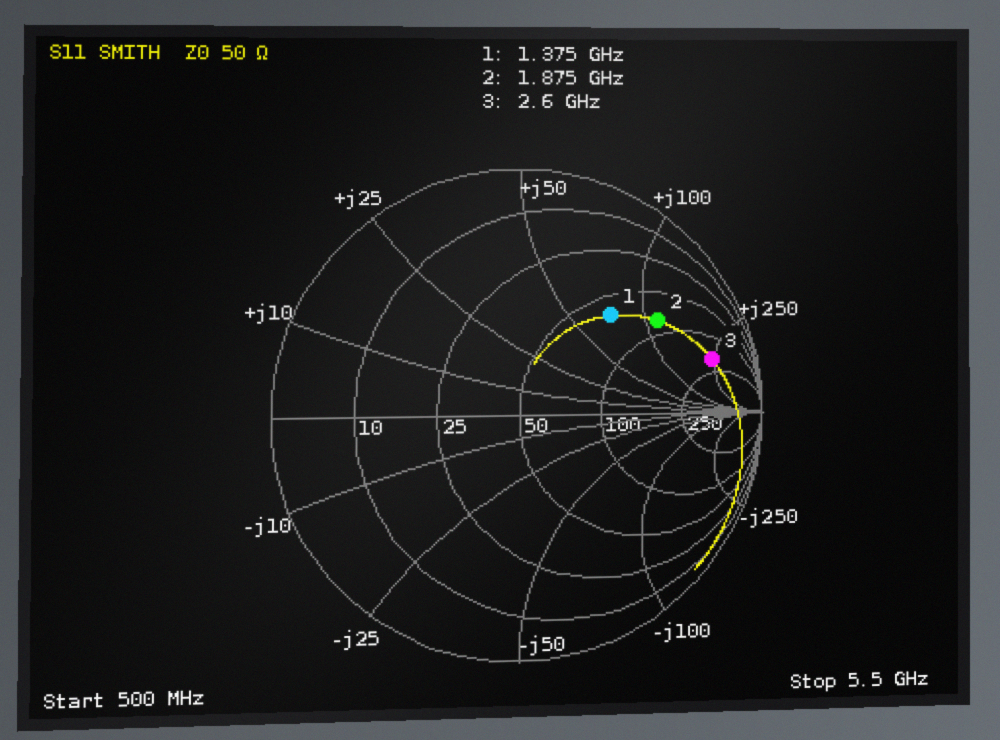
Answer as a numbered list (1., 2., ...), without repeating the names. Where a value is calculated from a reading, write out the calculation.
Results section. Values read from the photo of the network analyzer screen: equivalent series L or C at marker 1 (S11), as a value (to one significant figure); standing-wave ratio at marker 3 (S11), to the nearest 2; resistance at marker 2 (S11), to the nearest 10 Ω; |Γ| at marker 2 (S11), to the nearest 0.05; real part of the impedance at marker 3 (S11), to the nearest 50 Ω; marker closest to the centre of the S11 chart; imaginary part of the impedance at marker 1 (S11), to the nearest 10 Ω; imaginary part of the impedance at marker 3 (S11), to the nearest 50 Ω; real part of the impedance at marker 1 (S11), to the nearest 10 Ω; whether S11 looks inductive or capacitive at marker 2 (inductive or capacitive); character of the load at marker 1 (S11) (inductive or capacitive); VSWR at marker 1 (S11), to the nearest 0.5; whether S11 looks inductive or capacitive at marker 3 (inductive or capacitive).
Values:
1. L = 70 Ω/(2π × 1.375 GHz) ≈ 8 nH
2. 10
3. 80 Ω
4. 0.70
5. 200 Ω
6. marker 1
7. +70 Ω
8. +250 Ω
9. 60 Ω
10. inductive
11. inductive
12. 3.5
13. inductive
